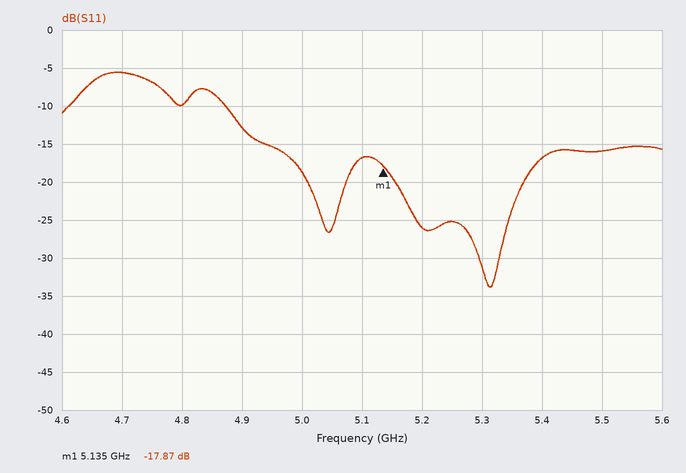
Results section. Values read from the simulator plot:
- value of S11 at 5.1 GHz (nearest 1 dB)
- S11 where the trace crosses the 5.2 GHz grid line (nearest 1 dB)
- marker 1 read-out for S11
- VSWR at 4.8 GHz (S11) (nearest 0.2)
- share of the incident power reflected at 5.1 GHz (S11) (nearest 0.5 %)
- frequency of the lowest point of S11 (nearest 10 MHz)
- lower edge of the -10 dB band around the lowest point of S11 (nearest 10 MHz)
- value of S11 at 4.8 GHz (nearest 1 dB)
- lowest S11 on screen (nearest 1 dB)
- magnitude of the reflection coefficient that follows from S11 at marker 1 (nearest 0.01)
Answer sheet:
-17 dB
-26 dB
-17.87 dB
2.0
2.0 %
5.31 GHz
4.87 GHz
-10 dB
-34 dB
0.13
